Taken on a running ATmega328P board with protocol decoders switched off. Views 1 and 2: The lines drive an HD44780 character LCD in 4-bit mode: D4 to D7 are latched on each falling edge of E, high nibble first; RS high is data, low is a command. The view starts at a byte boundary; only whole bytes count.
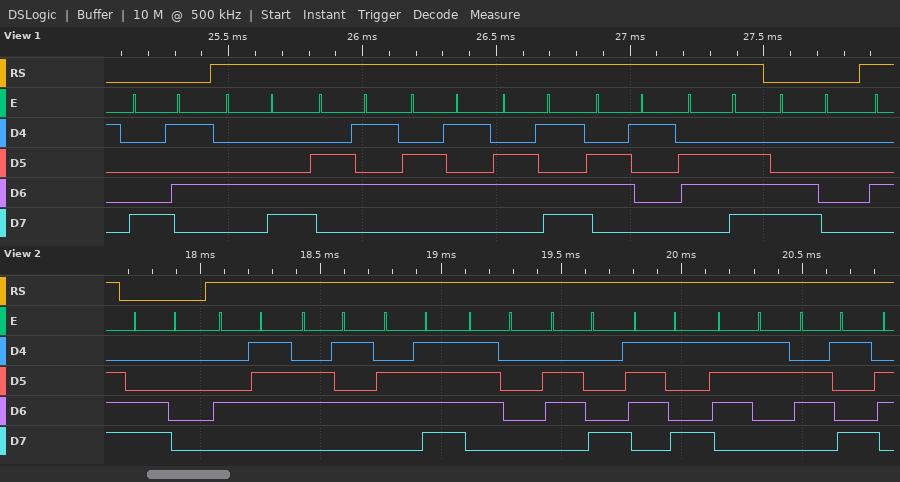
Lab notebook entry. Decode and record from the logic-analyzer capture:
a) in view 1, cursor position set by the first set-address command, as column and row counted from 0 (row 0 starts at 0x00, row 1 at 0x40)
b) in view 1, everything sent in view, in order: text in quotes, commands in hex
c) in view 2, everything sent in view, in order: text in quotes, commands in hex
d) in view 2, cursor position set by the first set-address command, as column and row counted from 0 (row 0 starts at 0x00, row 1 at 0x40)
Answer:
column 5, row 0
0x85 "Leeman" 0xC0
0xC0 "Geophysi"
column 0, row 1
